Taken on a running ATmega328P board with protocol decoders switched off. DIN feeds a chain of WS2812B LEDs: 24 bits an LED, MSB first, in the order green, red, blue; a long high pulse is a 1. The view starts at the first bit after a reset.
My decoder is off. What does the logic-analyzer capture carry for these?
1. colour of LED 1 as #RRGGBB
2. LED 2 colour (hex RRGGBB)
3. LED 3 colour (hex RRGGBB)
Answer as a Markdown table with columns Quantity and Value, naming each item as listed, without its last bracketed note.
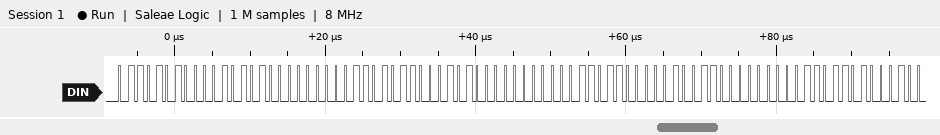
| Quantity | Value |
|---|---|
| colour of LED 1 as #RRGGBB | #156A00 |
| LED 2 colour | #146B00 |
| LED 3 colour | #136C00 |
